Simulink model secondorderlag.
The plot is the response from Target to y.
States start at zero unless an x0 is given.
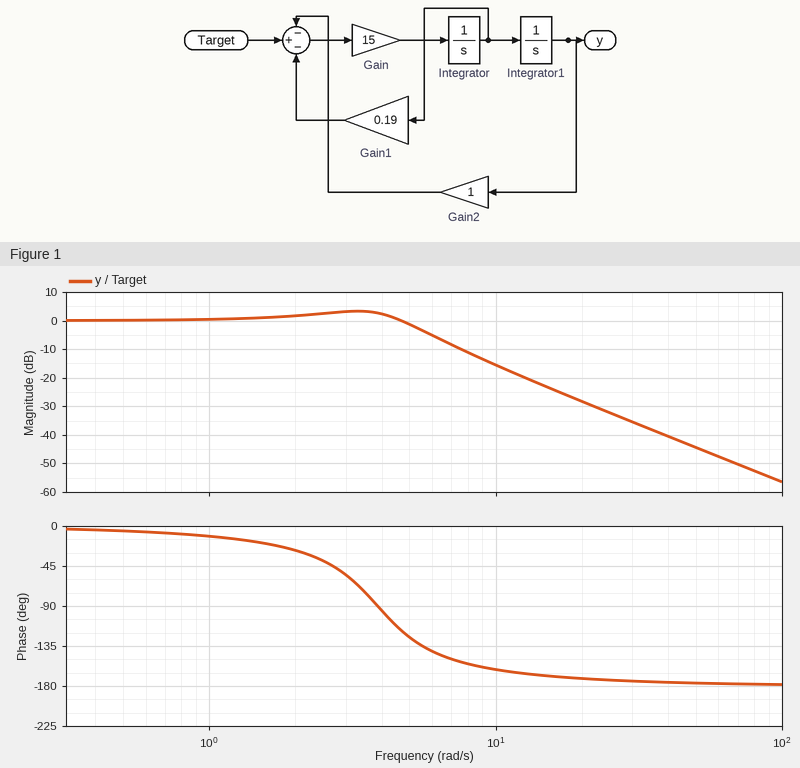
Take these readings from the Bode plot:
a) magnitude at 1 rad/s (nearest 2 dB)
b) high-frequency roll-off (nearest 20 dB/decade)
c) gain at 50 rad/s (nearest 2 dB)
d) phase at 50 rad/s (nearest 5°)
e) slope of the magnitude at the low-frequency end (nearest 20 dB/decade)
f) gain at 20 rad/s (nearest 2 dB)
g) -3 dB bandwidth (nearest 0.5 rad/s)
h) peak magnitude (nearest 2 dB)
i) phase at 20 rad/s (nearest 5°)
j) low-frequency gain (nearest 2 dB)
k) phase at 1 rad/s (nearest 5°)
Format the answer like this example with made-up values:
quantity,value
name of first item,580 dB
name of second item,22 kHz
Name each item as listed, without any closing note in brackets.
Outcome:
quantity,value
magnitude at 1 rad/s,0 dB
high-frequency roll-off,-40 dB/decade
gain at 50 rad/s,-44 dB
phase at 50 rad/s,-175°
slope of the magnitude at the low-frequency end,0 dB/decade
gain at 20 rad/s,-28 dB
-3 dB bandwidth,5.5 rad/s
peak magnitude,4 dB
phase at 20 rad/s,-170°
low-frequency gain,0 dB
phase at 1 rad/s,-10°
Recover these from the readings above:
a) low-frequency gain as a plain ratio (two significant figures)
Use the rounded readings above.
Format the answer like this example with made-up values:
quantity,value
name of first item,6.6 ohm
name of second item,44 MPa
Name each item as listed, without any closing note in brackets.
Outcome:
quantity,value
low-frequency gain as a plain ratio,1.0
